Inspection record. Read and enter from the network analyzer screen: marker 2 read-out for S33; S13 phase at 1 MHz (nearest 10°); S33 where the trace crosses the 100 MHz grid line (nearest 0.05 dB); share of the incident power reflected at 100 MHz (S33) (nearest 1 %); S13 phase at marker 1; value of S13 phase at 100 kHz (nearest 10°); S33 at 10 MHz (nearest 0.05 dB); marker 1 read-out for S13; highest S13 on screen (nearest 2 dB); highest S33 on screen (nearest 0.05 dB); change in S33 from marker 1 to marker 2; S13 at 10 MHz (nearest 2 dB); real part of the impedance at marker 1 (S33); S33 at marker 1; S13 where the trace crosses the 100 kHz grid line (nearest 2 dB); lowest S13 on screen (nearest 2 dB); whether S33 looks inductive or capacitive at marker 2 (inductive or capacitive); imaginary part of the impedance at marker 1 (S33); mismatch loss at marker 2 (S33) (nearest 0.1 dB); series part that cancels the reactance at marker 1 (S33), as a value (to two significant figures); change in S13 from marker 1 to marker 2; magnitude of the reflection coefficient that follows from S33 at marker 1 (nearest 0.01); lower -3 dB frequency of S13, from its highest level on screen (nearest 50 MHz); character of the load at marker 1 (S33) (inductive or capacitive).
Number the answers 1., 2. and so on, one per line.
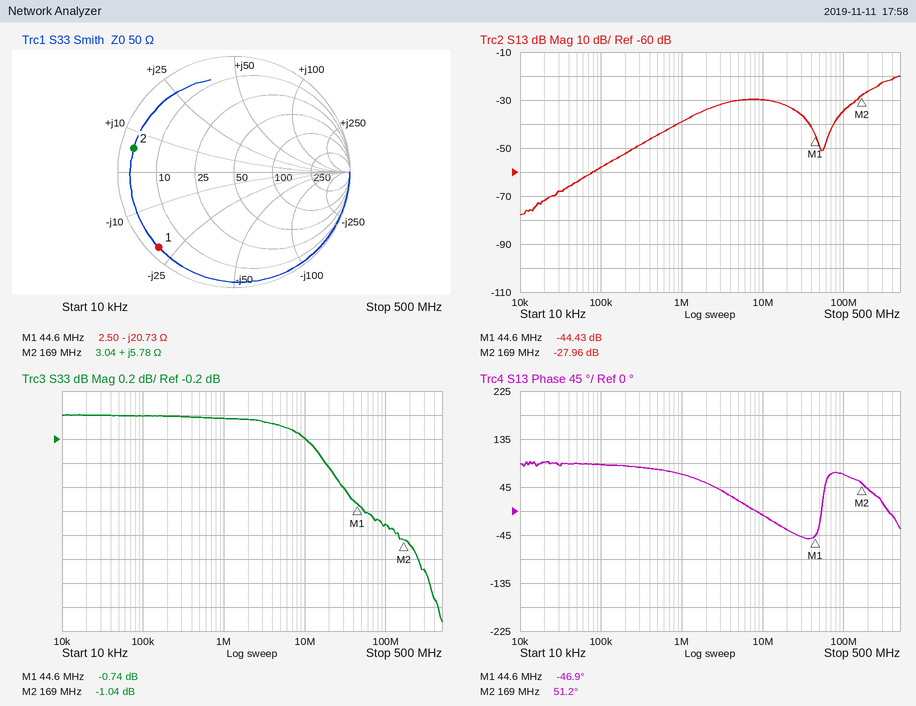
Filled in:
1. -1.04 dB
2. 70°
3. -0.90 dB
4. 81 %
5. -46.9°
6. 90°
7. -0.20 dB
8. -44.43 dB
9. -20 dB
10. 0.00 dB
11. -0.30 dB
12. -30 dB
13. 2.50 Ω
14. -0.74 dB
15. -58 dB
16. -78 dB
17. inductive
18. -20.73 Ω
19. 6.7 dB
20. 74 nH
21. 16.47 dB
22. 0.92
23. 300 MHz
24. capacitive
